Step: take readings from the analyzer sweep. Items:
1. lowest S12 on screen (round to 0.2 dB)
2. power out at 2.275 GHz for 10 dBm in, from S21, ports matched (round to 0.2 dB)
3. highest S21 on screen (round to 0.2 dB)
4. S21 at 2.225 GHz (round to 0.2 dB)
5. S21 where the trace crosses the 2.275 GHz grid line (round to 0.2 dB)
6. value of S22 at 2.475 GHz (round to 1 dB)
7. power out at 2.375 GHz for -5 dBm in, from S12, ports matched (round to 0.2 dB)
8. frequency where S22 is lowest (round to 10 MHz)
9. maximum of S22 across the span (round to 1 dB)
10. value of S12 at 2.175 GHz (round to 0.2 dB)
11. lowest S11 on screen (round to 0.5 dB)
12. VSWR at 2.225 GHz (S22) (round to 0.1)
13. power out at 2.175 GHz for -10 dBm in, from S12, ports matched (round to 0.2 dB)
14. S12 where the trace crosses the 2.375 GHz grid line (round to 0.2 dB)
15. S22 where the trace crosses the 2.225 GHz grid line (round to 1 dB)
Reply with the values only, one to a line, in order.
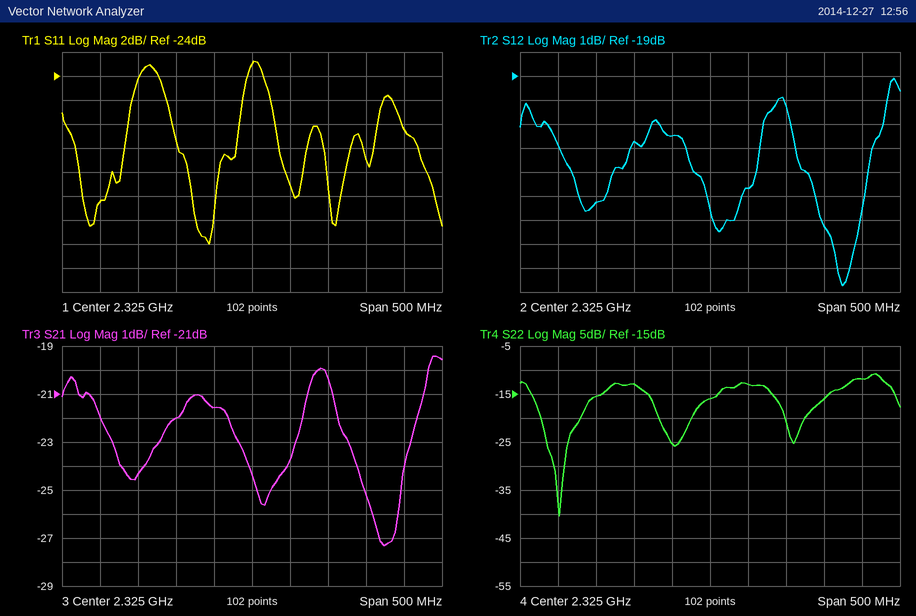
-27.8 dB
-11.6 dBm
-19.4 dB
-22.0 dB
-21.6 dB
-16 dB
-28.6 dBm
2.13 GHz
-11 dB
-24.2 dB
-38.0 dB
1.6
-34.2 dBm
-23.6 dB
-13 dB
